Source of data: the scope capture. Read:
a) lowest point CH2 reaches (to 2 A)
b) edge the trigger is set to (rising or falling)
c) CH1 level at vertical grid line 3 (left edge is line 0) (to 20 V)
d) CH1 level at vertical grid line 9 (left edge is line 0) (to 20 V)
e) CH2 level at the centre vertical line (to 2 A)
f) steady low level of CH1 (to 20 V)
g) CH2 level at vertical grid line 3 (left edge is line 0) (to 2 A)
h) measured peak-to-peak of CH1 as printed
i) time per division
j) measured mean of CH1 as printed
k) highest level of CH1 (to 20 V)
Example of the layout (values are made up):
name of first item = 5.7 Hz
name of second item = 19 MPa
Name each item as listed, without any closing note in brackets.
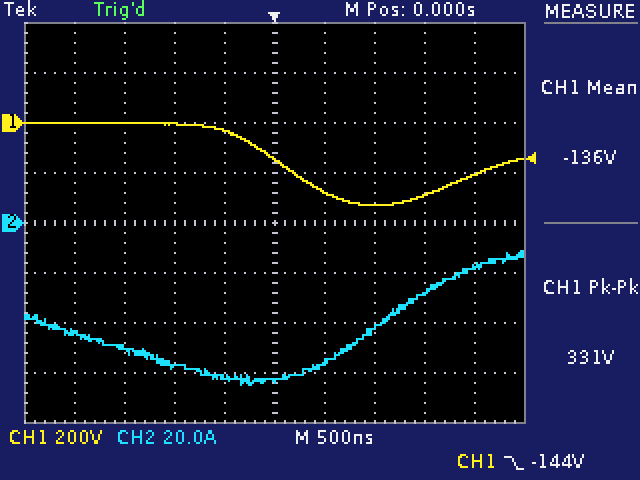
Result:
lowest point CH2 reaches = -64 A
edge the trigger is set to = falling
CH1 level at vertical grid line 3 (left edge is line 0) = 0 V
CH1 level at vertical grid line 9 (left edge is line 0) = -200 V
CH2 level at the centre vertical line = -64 A
steady low level of CH1 = -320 V
CH2 level at vertical grid line 3 (left edge is line 0) = -58 A
measured peak-to-peak of CH1 as printed = 331 V
time per division = 500 ns
measured mean of CH1 as printed = -136 V
highest level of CH1 = 0 V
